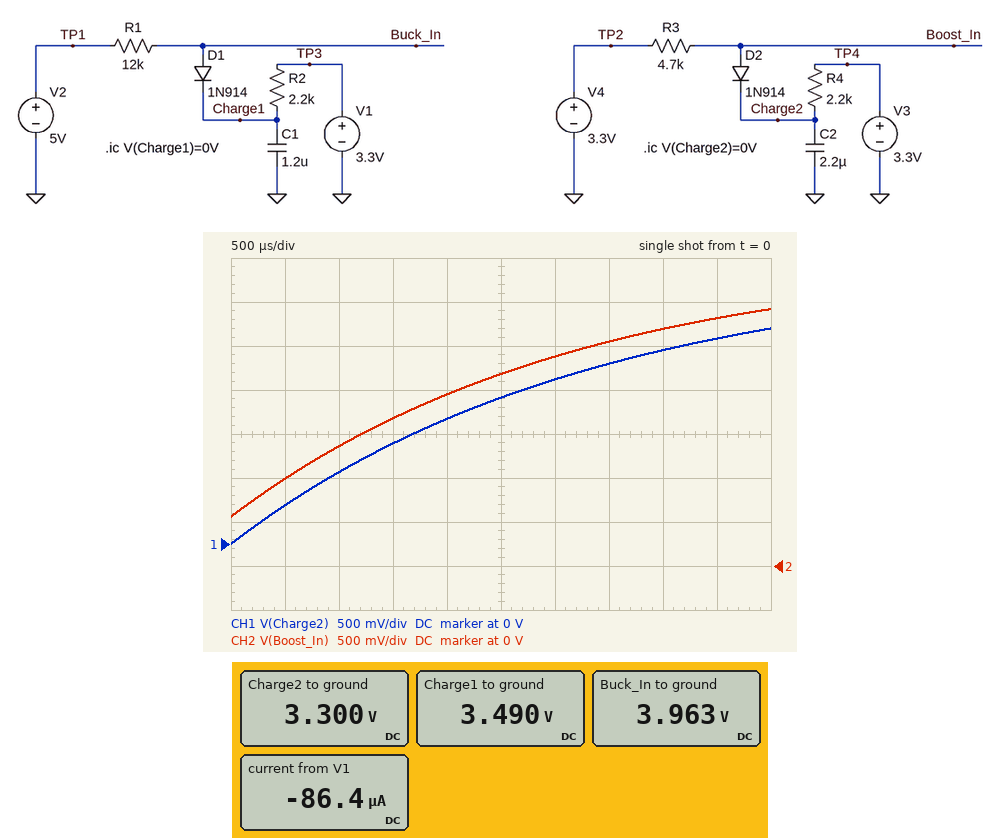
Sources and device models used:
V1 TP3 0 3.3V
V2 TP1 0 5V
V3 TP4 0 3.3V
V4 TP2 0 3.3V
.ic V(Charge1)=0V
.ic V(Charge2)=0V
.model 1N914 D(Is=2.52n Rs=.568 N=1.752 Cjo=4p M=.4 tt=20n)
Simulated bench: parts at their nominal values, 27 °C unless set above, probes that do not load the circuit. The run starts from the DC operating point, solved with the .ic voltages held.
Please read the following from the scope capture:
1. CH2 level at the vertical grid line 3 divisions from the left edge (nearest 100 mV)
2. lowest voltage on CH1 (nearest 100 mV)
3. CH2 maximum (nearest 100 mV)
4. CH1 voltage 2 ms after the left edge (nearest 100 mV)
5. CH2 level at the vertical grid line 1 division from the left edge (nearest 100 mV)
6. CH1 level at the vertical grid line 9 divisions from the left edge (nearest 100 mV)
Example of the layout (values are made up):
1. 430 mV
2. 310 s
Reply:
1. 1.7 V
2. 0 V
3. 2.9 V
4. 1.4 V
5. 1.0 V
6. 2.3 V
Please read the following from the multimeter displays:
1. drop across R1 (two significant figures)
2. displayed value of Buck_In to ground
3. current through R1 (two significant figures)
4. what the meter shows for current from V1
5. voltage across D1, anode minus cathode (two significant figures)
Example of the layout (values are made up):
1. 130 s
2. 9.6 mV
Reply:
1. 1.0 V
2. 3.963 V
3. 86 µA
4. -86.4 µA
5. 470 mV
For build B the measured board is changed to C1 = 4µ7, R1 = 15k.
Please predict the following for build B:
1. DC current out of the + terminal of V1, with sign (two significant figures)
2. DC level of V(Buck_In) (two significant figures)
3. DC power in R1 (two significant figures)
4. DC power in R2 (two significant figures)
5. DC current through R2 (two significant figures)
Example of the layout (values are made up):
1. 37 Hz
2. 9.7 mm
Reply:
1. -72 µA
2. 3.9 V
3. 77 µW
4. 11 µW
5. 72 µA
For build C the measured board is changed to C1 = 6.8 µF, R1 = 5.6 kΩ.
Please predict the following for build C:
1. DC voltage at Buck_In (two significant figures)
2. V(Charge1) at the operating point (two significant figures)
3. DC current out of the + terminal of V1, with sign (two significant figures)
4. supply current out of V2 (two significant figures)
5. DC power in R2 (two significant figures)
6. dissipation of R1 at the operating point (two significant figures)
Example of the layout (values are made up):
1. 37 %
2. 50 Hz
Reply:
1. 4.1 V
2. 3.6 V
3. -150 µA
4. 150 µA
5. 52 µW
6. 130 µW
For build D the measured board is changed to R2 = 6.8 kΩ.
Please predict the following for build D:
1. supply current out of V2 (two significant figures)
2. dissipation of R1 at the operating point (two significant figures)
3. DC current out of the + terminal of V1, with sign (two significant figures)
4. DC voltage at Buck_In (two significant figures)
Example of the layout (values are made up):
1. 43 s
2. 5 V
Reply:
1. 66 µA
2. 52 µW
3. -66 µA
4. 4.2 V
